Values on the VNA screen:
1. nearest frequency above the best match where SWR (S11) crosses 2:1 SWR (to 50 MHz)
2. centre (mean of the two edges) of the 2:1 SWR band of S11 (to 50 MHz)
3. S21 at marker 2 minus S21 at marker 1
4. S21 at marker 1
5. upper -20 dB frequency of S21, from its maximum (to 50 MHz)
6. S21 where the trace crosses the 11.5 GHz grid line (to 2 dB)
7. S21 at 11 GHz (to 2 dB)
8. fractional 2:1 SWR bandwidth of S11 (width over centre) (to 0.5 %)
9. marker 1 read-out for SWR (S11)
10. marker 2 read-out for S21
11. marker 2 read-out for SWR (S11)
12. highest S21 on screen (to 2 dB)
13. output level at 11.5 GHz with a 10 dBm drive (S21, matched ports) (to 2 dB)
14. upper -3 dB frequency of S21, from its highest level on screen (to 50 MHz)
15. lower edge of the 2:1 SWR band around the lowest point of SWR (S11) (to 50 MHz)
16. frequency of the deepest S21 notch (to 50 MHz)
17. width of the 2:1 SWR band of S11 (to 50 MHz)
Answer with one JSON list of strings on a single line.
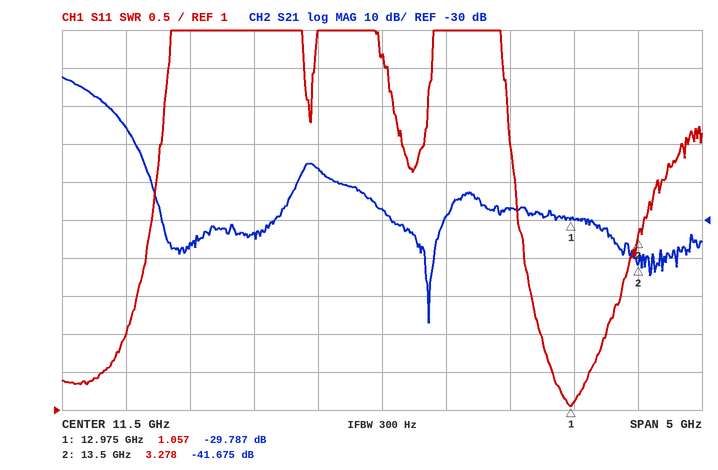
["13.25 GHz", "13.00 GHz", "-11.888 dB", "-29.787 dB", "9.60 GHz", "-28 dB", "-16 dB", "4.0 %", "1.057", "-41.675 dB", "3.278", "8 dB", "-18 dBm", "9.15 GHz", "12.75 GHz", "11.85 GHz", "500 MHz"]
